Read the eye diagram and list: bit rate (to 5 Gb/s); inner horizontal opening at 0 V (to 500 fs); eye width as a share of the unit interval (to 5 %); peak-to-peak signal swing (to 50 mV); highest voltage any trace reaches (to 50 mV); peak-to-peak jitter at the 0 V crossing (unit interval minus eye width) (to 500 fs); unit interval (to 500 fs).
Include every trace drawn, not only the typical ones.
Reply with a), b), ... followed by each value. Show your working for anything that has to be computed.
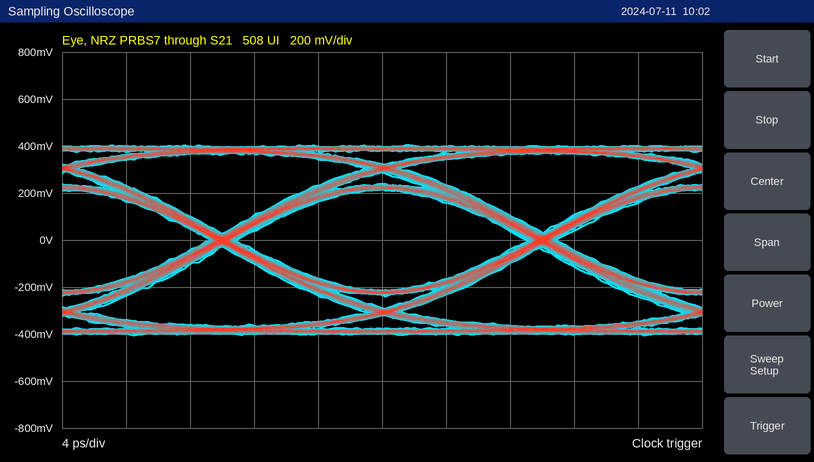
a) 50 Gb/s
b) 18.0 ps
c) 18.0 ps / 20.0 ps ≈ 90 %
d) 800 mV
e) 400 mV
f) 2.0 ps
g) 20.0 ps
